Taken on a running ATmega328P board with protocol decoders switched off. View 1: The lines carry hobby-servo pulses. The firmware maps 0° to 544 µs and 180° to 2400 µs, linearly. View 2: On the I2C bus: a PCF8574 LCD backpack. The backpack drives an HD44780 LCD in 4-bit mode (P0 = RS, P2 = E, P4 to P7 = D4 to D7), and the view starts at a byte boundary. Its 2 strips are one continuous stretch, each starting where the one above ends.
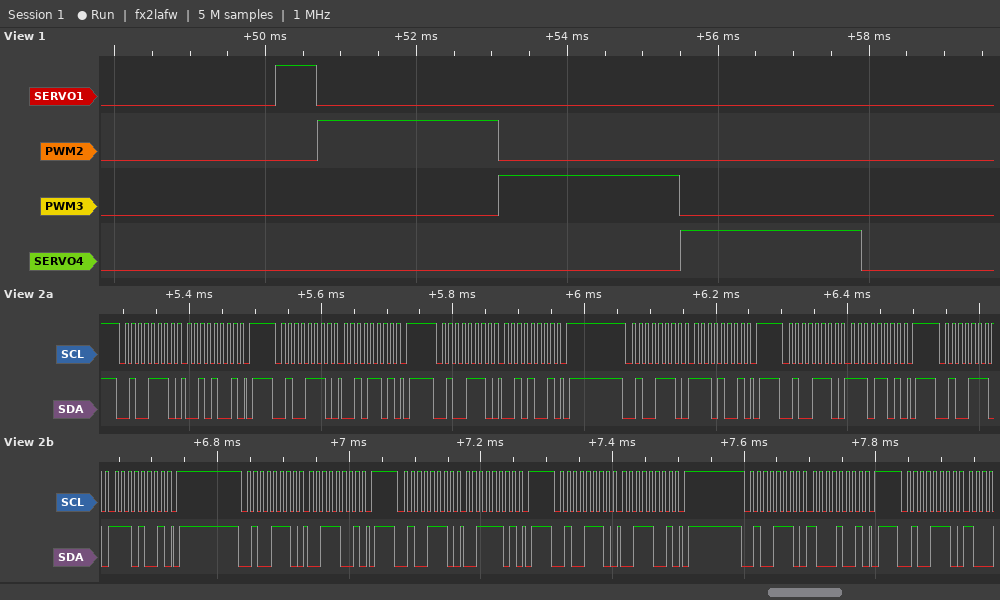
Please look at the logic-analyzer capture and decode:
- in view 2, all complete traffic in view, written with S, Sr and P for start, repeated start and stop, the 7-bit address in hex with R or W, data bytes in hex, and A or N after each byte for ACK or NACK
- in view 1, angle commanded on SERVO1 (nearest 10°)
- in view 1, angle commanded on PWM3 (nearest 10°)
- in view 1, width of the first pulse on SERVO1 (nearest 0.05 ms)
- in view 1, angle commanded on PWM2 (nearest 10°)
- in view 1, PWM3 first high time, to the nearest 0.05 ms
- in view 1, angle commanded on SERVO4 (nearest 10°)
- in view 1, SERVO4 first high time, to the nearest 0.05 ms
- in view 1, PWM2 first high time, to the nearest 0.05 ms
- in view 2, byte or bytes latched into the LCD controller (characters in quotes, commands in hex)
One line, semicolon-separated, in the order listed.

S 27W A 29 A P S 27W A 2D A P S 27W A 29 A P S 27W A E9 A P S 27W A ED A P S 27W A E9 A P S 27W A 39 A P S 27W A 3D A P S 27W A 39 A P S 27W A 89 A P S 27W A; 0°; 180°; 0.55 ms; 180°; 2.40 ms; 180°; 2.40 ms; 2.40 ms; '.'
